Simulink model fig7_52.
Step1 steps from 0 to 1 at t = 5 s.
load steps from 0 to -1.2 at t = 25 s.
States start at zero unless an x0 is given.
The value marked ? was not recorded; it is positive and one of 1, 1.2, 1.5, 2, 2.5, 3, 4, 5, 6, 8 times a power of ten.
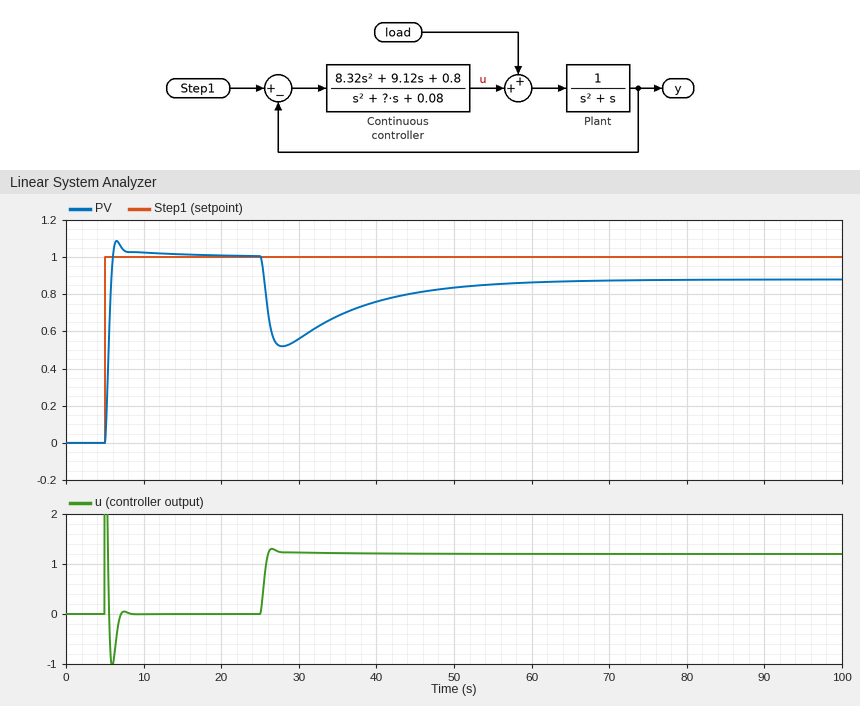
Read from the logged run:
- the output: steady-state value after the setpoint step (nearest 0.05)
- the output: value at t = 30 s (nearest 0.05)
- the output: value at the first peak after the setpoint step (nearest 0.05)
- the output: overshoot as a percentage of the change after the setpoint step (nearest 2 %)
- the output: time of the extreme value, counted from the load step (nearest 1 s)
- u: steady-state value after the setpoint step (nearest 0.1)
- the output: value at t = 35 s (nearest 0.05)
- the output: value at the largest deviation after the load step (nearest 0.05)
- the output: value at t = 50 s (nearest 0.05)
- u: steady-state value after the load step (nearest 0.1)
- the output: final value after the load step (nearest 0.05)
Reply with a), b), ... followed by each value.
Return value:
a) 1.00
b) 0.55
c) 1.10
d) 8 %
e) 3 s
f) 0.0
g) 0.70
h) 0.50
i) 0.85
j) 1.2
k) 0.90
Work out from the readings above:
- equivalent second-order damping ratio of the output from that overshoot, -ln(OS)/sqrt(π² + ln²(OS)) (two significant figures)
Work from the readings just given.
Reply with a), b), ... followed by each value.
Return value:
a) 0.63
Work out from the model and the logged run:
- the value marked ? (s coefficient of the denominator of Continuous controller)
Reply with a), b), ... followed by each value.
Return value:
a) 4
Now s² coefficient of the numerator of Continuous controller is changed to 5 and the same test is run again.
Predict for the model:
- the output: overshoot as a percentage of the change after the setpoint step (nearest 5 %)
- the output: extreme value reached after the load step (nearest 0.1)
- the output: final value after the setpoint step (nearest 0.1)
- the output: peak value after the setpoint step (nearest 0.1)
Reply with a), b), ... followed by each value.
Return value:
a) 20 %
b) 0.4
c) 1.0
d) 1.2
